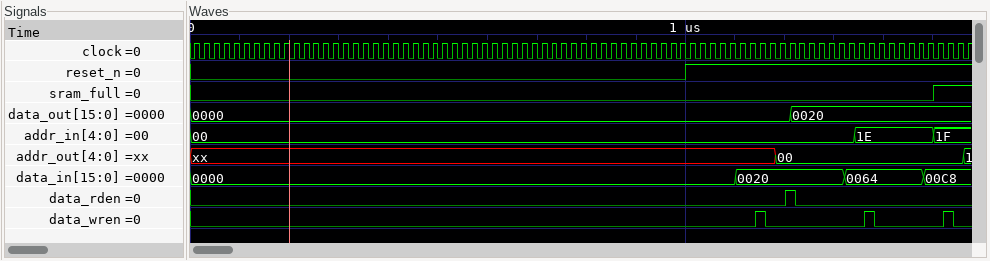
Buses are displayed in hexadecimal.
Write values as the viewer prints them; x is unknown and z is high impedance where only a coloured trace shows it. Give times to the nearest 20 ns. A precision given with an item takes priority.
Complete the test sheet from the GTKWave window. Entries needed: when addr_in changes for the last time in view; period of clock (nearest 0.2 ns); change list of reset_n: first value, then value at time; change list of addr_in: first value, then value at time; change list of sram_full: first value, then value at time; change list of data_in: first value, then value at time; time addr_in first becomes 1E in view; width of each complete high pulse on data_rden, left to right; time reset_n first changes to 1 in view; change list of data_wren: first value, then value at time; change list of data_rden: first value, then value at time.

1500 ns
20 ns
0, 1 at 1000 ns
00, 1E at 1340 ns, 1F at 1500 ns
0, 1 at 1500 ns
0000, 0020 at 1100 ns, 0064 at 1320 ns, 00C8 at 1480 ns
1340 ns
20 ns
1000 ns
0, 1 at 1140 ns, 0 at 1160 ns, 1 at 1360 ns, 0 at 1380 ns, 1 at 1520 ns, 0 at 1540 ns
0, 1 at 1200 ns, 0 at 1220 ns
